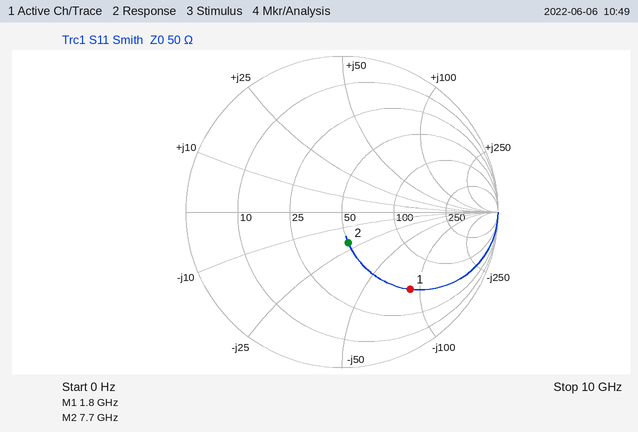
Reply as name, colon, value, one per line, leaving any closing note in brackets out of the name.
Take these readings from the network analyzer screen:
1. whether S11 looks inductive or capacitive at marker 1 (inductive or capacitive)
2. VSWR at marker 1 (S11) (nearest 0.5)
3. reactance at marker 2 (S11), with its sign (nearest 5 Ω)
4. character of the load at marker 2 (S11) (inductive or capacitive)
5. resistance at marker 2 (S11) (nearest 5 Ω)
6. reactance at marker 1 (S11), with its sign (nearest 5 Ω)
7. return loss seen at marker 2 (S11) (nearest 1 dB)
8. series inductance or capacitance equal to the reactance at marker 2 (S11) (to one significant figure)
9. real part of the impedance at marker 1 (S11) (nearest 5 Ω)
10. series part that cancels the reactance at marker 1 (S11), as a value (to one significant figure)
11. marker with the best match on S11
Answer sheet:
whether S11 looks inductive or capacitive at marker 1: capacitive
VSWR at marker 1 (S11): 5.0
reactance at marker 2 (S11), with its sign: -20 Ω
character of the load at marker 2 (S11): capacitive
resistance at marker 2 (S11): 50 Ω
reactance at marker 1 (S11), with its sign: -90 Ω
return loss seen at marker 2 (S11): 14 dB
series inductance or capacitance equal to the reactance at marker 2 (S11): 1.0 pF
real part of the impedance at marker 1 (S11): 50 Ω
series part that cancels the reactance at marker 1 (S11), as a value: 8 nH
marker with the best match on S11: marker 2
